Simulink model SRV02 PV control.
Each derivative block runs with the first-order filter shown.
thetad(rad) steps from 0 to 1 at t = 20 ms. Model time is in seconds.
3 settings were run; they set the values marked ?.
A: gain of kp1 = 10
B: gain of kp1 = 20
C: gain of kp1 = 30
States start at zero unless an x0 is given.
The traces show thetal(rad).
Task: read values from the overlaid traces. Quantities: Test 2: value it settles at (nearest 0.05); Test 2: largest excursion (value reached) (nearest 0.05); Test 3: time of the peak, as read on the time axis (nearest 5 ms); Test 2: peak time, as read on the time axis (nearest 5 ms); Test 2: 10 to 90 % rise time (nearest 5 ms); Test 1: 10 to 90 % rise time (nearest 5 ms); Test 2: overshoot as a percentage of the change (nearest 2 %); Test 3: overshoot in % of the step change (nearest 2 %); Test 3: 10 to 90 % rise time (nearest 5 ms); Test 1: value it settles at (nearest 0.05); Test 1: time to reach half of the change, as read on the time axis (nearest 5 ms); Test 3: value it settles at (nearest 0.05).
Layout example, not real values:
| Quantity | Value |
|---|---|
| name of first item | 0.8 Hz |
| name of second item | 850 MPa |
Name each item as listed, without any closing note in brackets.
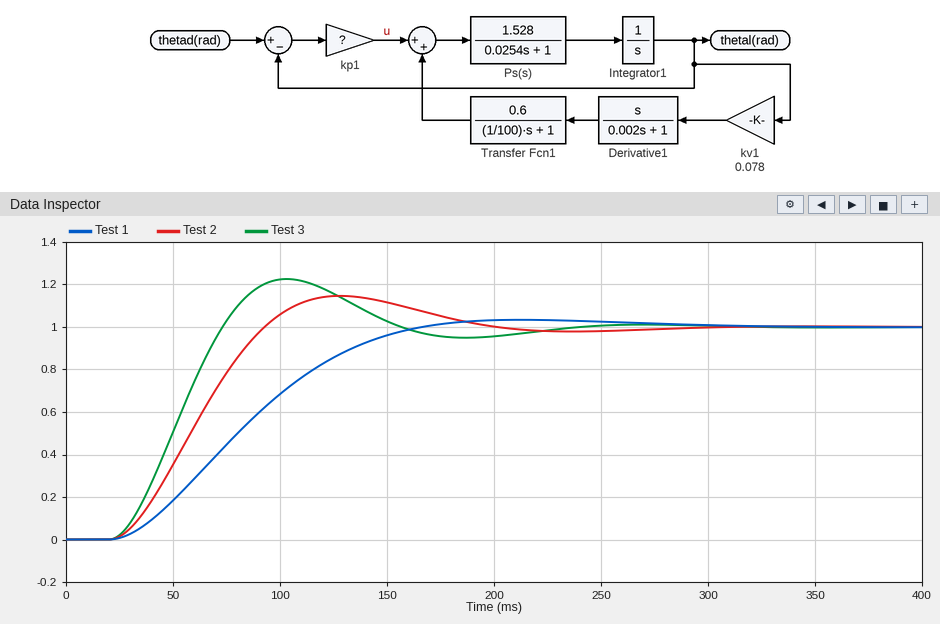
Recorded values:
| Quantity | Value |
|---|---|
| Test 2: value it settles at | 1.00 |
| Test 2: largest excursion (value reached) | 1.15 |
| Test 3: time of the peak, as read on the time axis | 105 ms |
| Test 2: peak time, as read on the time axis | 130 ms |
| Test 2: 10 to 90 % rise time | 50 ms |
| Test 1: 10 to 90 % rise time | 95 ms |
| Test 2: overshoot as a percentage of the change | 14 % |
| Test 3: overshoot in % of the step change | 22 % |
| Test 3: 10 to 90 % rise time | 35 ms |
| Test 1: value it settles at | 1.00 |
| Test 1: time to reach half of the change, as read on the time axis | 80 ms |
| Test 3: value it settles at | 1.00 |
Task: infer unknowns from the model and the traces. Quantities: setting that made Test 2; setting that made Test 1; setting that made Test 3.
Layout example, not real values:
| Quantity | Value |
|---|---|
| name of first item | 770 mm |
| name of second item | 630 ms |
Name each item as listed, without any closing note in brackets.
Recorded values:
| Quantity | Value |
|---|---|
| setting that made Test 2 | B |
| setting that made Test 1 | A |
| setting that made Test 3 | C |
